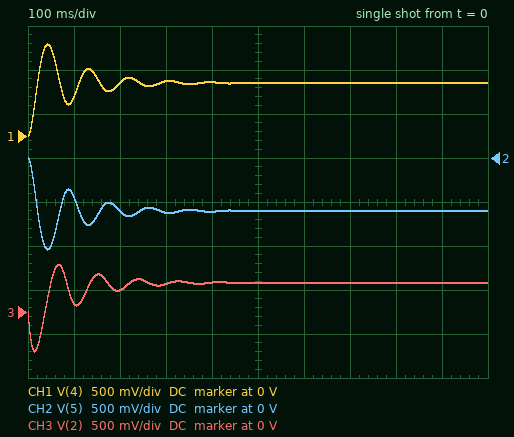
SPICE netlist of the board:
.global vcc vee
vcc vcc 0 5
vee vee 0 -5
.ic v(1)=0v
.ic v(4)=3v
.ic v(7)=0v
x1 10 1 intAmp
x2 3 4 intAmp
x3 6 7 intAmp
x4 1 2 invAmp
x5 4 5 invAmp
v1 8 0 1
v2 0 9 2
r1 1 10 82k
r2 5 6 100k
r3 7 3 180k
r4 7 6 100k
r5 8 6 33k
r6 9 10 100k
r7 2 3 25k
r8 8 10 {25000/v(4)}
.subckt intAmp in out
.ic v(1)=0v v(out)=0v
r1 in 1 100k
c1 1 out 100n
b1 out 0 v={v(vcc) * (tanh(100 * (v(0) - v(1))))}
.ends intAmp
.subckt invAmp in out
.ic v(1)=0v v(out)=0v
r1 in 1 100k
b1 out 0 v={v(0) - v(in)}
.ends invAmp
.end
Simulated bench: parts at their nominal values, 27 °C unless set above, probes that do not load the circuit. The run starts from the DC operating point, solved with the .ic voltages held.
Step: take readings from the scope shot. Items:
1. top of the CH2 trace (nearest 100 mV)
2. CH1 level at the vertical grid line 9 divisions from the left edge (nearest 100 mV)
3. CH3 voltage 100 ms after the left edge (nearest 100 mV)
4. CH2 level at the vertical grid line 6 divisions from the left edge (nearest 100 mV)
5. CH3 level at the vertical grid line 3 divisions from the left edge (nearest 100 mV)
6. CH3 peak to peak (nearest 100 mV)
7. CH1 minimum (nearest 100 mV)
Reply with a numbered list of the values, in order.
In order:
1. 0 V
2. 600 mV
3. 100 mV
4. -600 mV
5. 300 mV
6. 1.0 V
7. 0 V
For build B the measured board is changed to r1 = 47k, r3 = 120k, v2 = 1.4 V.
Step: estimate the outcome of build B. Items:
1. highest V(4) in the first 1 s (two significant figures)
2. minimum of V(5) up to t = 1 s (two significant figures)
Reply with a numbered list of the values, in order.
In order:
1. 800 mV
2. -800 mV
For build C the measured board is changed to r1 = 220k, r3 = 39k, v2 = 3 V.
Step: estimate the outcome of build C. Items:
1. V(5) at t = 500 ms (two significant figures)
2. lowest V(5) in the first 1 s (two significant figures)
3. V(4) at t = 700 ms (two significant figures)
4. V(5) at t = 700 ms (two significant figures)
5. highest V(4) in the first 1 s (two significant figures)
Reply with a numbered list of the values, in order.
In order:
1. -790 mV
2. -2.3 V
3. 860 mV
4. -860 mV
5. 2.3 V
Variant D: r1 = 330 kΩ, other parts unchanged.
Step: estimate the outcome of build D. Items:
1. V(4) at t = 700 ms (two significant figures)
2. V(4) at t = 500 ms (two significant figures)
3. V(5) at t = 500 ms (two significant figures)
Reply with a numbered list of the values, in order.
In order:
1. 480 mV
2. 630 mV
3. -630 mV
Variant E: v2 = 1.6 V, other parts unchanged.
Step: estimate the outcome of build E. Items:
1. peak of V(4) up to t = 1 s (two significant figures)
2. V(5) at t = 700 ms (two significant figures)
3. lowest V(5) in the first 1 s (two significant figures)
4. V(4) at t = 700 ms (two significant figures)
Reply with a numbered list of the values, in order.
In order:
1. 840 mV
2. -510 mV
3. -840 mV
4. 510 mV
